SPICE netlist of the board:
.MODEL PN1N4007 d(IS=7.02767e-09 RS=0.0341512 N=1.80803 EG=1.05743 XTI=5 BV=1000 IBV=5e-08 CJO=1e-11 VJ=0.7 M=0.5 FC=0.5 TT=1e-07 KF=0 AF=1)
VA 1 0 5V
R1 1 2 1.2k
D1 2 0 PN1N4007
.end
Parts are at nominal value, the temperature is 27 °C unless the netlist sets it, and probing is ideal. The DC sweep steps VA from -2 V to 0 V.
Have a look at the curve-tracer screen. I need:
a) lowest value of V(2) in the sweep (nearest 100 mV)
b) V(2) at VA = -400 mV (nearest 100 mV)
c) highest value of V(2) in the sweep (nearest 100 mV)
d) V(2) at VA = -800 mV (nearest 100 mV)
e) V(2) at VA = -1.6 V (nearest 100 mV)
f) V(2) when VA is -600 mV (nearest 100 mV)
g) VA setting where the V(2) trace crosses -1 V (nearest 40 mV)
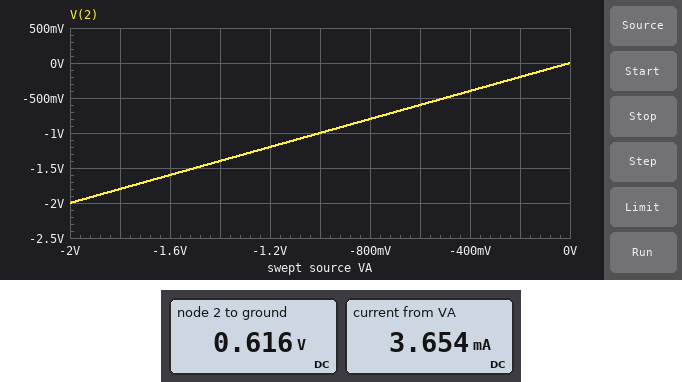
-2.0 V
-400 mV
0 V
-800 mV
-1.6 V
-600 mV
-1.00 V
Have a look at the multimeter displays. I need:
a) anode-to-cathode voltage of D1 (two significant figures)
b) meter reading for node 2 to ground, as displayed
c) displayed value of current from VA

620 mV
0.616 V
3.654 mA
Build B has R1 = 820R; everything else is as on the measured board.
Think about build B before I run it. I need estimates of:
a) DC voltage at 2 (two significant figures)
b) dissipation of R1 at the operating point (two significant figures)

630 mV
23 mW
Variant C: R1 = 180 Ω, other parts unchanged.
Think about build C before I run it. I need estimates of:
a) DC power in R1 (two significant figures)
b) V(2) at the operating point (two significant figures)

100 mW
700 mV
